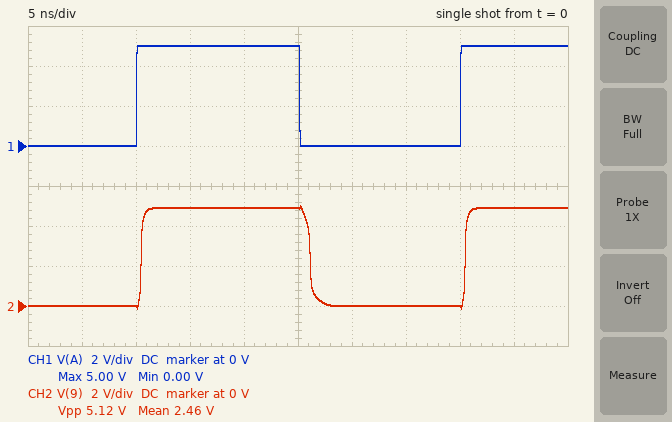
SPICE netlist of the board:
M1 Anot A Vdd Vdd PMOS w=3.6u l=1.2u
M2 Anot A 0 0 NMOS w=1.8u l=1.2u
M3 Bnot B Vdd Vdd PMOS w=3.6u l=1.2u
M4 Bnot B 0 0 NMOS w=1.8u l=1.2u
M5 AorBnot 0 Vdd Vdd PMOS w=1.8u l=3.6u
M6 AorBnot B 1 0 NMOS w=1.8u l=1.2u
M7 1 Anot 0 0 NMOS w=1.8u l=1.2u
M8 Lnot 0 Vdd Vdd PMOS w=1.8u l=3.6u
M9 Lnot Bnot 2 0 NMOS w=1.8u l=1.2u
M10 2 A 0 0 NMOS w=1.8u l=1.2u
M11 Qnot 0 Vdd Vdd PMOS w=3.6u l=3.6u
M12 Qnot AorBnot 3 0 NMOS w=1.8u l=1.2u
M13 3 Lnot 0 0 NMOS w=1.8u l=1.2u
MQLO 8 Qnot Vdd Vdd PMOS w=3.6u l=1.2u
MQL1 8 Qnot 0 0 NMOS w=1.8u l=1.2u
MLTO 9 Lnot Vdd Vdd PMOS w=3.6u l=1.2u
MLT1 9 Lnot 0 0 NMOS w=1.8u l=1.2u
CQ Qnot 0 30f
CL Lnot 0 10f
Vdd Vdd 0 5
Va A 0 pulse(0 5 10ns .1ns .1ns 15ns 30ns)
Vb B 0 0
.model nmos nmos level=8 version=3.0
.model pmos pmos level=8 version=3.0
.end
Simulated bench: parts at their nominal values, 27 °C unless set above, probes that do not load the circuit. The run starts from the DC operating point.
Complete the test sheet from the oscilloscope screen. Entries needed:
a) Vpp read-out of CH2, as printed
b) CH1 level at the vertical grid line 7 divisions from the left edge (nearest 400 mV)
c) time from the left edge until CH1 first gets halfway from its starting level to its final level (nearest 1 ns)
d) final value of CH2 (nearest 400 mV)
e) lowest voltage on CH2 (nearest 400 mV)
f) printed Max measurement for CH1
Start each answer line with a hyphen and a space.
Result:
- 5.12 V
- 0 V
- 10 ns
- 4.8 V
- 0 V
- 5.00 V
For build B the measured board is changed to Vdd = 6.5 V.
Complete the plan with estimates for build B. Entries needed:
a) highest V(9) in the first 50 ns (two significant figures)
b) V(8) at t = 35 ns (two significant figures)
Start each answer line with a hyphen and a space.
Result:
- 6.2 V
- 5.5 V
